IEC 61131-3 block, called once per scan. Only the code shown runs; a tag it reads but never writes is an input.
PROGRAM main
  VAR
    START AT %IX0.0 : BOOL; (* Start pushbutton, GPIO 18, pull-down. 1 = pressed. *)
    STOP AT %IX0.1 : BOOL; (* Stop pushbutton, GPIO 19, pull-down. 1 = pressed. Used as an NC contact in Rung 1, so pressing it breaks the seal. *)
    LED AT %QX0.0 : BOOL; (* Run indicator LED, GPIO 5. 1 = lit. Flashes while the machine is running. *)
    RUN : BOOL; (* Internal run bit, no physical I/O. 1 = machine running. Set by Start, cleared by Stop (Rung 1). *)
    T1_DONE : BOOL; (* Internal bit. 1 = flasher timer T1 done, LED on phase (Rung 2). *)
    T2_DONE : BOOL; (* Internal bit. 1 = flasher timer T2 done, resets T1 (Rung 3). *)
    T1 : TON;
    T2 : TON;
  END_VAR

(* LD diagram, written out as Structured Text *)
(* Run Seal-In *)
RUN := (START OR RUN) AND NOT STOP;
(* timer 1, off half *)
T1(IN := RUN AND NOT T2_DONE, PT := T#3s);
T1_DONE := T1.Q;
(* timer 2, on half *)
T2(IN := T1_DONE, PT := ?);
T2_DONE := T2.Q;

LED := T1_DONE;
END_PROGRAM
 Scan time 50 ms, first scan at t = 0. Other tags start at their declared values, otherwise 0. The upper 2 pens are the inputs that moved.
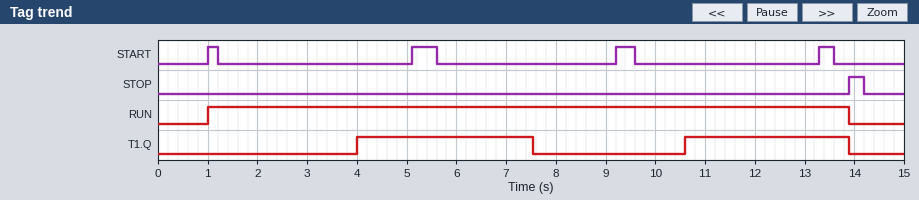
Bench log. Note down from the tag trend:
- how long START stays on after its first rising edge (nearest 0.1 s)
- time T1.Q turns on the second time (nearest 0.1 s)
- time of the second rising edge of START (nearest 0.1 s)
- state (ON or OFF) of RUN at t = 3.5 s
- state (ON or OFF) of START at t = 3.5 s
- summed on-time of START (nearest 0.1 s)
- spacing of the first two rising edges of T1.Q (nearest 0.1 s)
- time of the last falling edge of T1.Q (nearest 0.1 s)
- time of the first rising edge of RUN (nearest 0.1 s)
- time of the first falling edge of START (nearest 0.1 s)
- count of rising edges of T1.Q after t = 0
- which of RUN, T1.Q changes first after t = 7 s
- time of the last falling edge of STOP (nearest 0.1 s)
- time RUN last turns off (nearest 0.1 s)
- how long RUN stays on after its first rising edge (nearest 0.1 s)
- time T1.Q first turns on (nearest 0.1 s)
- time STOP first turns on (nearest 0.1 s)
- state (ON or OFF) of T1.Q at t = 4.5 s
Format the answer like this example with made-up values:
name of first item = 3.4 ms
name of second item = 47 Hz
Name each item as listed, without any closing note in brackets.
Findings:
how long START stays on after its first rising edge = 0.2 s
time T1.Q turns on the second time = 10.6 s
time of the second rising edge of START = 5.1 s
state (ON or OFF) of RUN at t = 3.5 s = ON
state (ON or OFF) of START at t = 3.5 s = OFF
summed on-time of START = 1.4 s
spacing of the first two rising edges of T1.Q = 6.6 s
time of the last falling edge of T1.Q = 13.9 s
time of the first rising edge of RUN = 1.0 s
time of the first falling edge of START = 1.2 s
count of rising edges of T1.Q after t = 0 = 2
which of RUN, T1.Q changes first after t = 7 s = T1.Q
time of the last falling edge of STOP = 14.2 s
time RUN last turns off = 13.9 s
how long RUN stays on after its first rising edge = 12.9 s
time T1.Q first turns on = 4.0 s
time STOP first turns on = 13.9 s
state (ON or OFF) of T1.Q at t = 4.5 s = ON
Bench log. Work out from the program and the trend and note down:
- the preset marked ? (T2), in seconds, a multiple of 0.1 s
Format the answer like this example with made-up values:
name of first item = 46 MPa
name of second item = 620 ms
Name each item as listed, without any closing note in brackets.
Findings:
the preset marked ? (T2), in seconds, a multiple of 0.1 s = 3.5 s
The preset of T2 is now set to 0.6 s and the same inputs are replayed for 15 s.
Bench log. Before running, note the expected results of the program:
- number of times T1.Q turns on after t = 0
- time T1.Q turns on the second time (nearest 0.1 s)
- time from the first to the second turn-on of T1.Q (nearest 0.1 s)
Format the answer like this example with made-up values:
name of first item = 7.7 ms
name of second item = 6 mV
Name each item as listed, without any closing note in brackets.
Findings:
number of times T1.Q turns on after t = 0 = 3
time T1.Q turns on the second time = 7.7 s
time from the first to the second turn-on of T1.Q = 3.7 s
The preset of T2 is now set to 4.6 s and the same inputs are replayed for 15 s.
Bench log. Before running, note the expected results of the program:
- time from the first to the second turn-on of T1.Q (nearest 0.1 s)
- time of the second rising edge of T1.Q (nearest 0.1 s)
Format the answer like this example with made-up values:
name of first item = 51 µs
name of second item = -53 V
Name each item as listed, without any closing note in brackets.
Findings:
time from the first to the second turn-on of T1.Q = 7.7 s
time of the second rising edge of T1.Q = 11.7 s
